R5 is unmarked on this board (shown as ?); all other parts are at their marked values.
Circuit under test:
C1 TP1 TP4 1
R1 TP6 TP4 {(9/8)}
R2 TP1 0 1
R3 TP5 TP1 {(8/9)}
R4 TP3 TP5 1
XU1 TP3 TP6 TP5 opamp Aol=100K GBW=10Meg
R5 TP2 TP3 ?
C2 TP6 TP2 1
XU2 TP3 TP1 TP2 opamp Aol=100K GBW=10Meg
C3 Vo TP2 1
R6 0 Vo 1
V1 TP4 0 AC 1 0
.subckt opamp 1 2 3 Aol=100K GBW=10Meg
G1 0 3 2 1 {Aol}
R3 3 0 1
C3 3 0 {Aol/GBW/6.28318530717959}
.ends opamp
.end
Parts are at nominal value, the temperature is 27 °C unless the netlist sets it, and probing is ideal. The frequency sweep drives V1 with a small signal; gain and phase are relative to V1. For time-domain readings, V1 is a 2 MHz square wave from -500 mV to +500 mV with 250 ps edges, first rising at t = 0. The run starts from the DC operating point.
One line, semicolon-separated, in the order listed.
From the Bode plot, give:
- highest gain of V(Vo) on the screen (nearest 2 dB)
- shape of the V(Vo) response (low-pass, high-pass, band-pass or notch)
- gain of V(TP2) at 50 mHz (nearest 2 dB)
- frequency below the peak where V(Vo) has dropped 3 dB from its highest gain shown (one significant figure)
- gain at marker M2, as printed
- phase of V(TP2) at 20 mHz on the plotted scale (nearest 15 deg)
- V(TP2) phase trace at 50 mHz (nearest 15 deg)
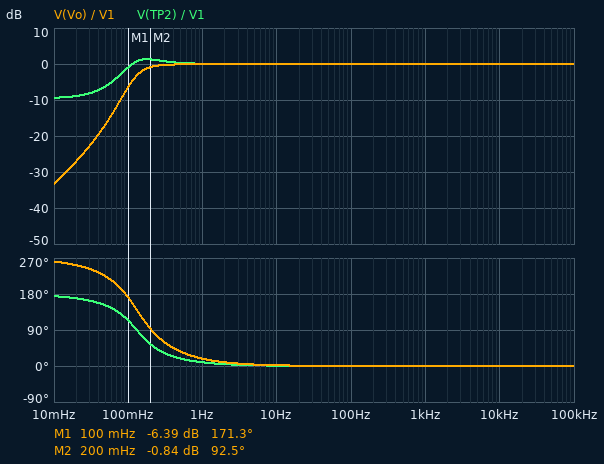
0 dB; high-pass; -6 dB; 100 mHz; -0.84 dB; 165 deg; 150 deg
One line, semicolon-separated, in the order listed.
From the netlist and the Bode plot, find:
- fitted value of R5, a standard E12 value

1.5 Ω
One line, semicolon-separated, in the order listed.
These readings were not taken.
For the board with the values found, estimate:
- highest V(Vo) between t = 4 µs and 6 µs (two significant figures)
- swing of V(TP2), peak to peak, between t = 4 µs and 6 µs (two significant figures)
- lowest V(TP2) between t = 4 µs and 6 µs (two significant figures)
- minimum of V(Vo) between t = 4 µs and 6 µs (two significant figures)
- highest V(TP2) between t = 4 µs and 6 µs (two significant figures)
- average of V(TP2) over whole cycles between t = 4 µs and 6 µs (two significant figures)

1.2 V; 1.5 V; -64 mV; -230 mV; 1.4 V; 670 mV
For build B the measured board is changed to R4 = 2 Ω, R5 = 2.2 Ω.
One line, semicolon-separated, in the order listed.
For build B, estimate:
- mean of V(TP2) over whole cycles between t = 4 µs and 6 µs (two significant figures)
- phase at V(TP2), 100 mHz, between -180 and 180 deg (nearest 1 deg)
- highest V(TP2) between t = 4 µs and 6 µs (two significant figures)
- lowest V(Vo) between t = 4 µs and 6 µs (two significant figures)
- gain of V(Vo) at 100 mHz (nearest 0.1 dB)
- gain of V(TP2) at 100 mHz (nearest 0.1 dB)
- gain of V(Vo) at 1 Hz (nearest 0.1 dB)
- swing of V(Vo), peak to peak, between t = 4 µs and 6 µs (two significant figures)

490 mV; 129 deg; 1.2 V; -210 mV; -12.2 dB; -6.7 dB; 0 dB; 1.4 V
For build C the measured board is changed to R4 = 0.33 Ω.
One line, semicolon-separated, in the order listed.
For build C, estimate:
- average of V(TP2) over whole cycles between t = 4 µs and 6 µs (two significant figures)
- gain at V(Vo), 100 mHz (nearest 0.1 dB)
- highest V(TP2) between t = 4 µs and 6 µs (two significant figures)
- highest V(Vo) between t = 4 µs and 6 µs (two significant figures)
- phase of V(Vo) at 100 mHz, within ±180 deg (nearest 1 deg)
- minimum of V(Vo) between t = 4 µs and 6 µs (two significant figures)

2.0 V; -1.2 dB; 2.8 V; 1.3 V; 132 deg; -270 mV
